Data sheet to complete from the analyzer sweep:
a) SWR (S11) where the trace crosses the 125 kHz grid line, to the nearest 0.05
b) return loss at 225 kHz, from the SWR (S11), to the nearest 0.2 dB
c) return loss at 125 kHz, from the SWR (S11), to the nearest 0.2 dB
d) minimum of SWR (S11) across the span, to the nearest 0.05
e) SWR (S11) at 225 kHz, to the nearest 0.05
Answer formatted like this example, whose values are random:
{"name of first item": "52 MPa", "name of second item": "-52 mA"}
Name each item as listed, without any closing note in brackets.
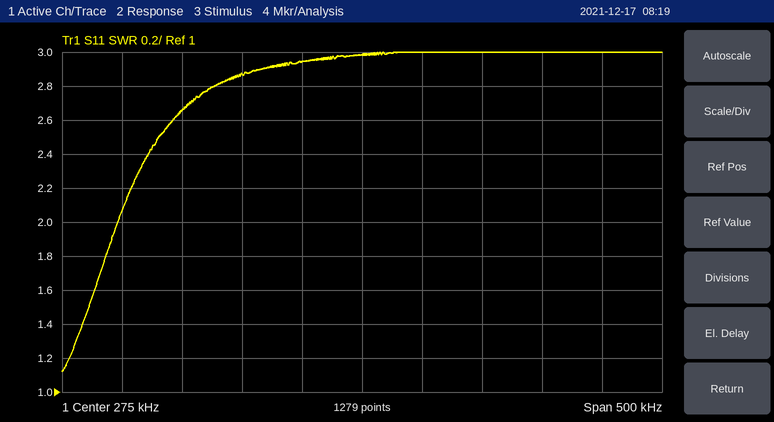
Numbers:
{"SWR (S11) where the trace crosses the 125 kHz grid line, to the nearest 0.05": "2.65", "return loss at 225 kHz, from the SWR (S11), to the nearest 0.2 dB": "6.2 dB", "return loss at 125 kHz, from the SWR (S11), to the nearest 0.2 dB": "6.8 dB", "minimum of SWR (S11) across the span, to the nearest 0.05": "1.10", "SWR (S11) at 225 kHz, to the nearest 0.05": "2.95"}
